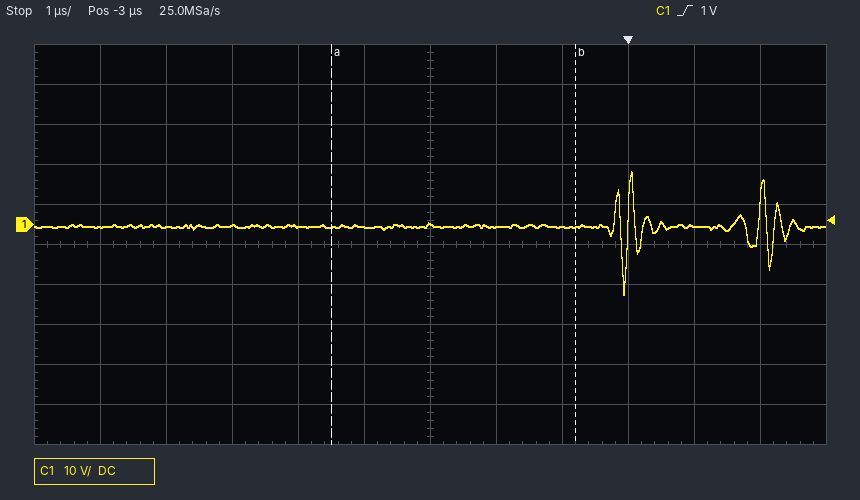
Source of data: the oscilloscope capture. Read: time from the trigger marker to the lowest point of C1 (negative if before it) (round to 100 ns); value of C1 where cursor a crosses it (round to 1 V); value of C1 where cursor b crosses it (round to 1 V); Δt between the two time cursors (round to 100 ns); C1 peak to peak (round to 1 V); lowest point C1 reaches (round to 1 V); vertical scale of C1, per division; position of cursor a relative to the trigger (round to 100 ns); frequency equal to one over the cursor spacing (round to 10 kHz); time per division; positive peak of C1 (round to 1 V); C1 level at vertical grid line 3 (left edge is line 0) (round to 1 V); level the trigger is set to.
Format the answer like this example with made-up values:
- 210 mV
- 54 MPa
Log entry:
- -100 ns
- -1 V
- -1 V
- 3.7 µs
- 31 V
- -18 V
- 10 V
- -4.5 µs
- 270 kHz
- 1 µs
- 13 V
- 0 V
- 1 V
